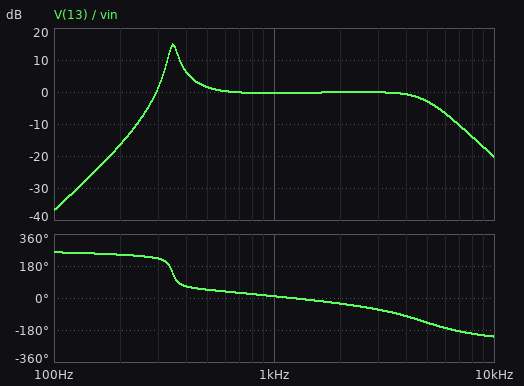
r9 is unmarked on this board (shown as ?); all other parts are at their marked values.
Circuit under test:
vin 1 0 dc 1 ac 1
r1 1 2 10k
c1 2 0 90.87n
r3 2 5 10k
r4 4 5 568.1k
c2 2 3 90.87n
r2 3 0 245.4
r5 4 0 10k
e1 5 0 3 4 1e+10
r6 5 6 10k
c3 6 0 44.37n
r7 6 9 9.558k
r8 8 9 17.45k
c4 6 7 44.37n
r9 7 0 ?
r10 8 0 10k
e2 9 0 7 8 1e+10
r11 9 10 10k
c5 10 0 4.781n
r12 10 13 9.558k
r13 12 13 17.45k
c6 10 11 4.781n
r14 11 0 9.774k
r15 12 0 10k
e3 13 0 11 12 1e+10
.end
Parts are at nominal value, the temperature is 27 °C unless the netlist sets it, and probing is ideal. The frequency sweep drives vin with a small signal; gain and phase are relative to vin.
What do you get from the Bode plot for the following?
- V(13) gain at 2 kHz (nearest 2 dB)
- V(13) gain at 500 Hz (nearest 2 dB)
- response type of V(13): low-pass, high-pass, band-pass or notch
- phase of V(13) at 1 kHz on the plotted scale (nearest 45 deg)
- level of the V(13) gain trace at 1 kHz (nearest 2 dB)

0 dB
2 dB
band-pass
0 deg
0 dB
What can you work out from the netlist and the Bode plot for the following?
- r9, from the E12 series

22 kΩ
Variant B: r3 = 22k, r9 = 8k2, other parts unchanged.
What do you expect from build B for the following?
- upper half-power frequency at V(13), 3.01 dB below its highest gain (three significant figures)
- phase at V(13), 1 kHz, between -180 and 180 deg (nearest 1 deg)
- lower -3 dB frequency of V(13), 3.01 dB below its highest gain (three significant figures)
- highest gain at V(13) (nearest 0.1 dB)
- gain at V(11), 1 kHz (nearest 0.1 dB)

5.48 kHz
35 deg
534 Hz
-6.1 dB
-15.6 dB
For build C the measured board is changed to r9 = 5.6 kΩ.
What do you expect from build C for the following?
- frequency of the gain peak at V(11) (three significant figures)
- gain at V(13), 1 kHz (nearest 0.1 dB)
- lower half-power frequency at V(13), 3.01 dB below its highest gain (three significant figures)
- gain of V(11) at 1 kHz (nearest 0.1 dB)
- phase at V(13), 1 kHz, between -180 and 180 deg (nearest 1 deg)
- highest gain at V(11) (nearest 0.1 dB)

2.91 kHz
-2.4 dB
878 Hz
-11.1 dB
70 deg
-9.0 dB
